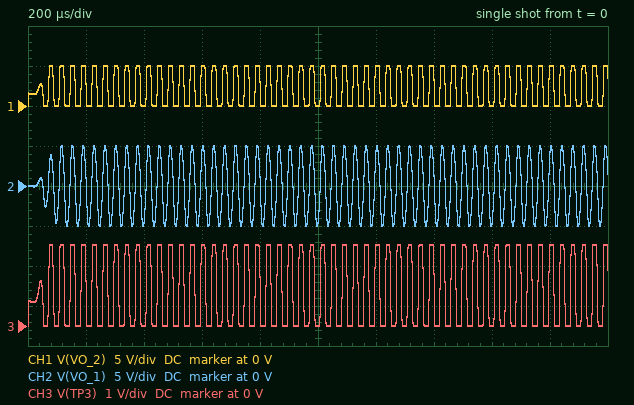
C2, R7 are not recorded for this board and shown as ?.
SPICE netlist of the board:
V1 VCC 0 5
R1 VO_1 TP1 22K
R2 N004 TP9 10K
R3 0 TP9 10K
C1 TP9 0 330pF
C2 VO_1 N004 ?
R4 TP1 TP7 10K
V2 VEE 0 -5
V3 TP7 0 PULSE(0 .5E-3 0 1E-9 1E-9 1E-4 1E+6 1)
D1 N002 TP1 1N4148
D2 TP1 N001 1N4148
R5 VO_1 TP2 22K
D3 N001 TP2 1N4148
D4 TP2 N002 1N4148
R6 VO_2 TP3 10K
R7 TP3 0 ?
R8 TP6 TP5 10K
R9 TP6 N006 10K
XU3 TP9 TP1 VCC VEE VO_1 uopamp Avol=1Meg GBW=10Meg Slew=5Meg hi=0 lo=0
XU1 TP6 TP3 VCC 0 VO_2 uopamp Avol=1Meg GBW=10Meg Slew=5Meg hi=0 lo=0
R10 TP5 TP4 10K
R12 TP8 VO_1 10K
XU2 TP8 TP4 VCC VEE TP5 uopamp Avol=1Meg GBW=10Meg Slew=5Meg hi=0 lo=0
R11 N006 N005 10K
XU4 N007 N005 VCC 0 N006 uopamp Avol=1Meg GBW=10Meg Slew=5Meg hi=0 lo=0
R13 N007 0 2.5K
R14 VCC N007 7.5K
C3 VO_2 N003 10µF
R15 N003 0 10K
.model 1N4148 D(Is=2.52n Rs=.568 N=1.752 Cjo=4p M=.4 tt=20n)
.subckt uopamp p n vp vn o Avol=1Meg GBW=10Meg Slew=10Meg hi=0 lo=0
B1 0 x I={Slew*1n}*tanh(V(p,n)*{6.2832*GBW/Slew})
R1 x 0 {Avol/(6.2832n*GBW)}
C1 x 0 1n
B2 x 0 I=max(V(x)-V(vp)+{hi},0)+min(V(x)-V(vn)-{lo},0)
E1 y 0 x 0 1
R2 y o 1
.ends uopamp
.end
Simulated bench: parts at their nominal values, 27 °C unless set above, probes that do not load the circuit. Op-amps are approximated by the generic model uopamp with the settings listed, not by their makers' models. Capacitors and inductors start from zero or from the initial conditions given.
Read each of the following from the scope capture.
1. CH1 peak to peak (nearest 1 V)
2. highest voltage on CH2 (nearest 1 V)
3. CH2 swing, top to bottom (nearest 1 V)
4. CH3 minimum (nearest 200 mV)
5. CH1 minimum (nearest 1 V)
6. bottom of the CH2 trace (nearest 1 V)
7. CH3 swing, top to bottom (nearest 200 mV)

5 V
5 V
10 V
0 V
0 V
-5 V
2.0 V
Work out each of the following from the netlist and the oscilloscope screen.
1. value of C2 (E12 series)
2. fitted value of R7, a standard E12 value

1 nF
6.8 kΩ
